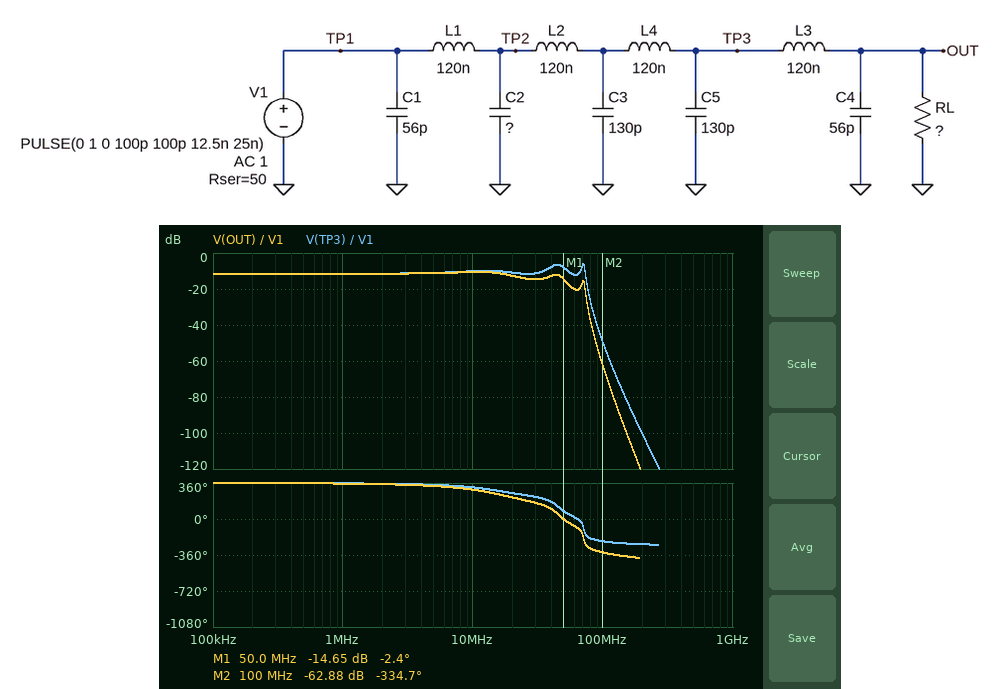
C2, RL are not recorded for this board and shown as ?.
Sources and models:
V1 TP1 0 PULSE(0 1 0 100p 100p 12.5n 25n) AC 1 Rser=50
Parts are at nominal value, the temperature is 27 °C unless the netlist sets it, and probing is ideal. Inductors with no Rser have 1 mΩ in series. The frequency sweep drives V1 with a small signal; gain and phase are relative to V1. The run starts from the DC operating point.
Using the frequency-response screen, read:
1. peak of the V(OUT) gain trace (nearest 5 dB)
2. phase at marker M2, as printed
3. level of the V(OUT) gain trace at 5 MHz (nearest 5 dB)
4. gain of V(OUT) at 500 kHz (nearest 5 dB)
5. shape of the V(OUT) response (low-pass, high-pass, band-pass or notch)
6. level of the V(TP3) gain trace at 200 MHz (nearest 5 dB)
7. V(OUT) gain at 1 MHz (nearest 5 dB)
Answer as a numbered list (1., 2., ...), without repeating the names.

1. -10 dB
2. -334.7 deg
3. -10 dB
4. -10 dB
5. low-pass
6. -100 dB
7. -10 dB
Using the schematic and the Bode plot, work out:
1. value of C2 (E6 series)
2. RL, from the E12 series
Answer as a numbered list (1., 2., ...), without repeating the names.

1. 330 pF
2. 18 Ω
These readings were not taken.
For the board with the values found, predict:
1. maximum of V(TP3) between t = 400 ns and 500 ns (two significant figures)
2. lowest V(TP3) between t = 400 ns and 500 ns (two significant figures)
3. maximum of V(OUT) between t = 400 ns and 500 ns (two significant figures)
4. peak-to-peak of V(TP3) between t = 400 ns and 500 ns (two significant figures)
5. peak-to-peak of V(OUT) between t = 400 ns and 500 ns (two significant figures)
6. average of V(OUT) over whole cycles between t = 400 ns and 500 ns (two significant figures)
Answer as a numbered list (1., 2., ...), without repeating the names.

1. 390 mV
2. -130 mV
3. 280 mV
4. 520 mV
5. 290 mV
6. 130 mV
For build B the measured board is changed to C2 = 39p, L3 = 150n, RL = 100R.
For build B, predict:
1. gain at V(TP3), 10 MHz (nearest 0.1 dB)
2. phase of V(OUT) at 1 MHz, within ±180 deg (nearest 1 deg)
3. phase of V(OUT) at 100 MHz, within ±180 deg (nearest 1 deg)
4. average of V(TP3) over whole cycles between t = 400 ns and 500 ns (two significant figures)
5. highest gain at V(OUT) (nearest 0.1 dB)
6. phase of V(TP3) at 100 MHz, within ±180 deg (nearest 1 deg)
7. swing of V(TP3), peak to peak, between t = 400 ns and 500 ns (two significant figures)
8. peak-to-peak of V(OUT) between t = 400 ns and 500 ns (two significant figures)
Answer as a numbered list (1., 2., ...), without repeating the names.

1. -4.7 dB
2. -6 deg
3. 134 deg
4. 340 mV
5. -3.1 dB
6. -68 deg
7. 460 mV
8. 780 mV
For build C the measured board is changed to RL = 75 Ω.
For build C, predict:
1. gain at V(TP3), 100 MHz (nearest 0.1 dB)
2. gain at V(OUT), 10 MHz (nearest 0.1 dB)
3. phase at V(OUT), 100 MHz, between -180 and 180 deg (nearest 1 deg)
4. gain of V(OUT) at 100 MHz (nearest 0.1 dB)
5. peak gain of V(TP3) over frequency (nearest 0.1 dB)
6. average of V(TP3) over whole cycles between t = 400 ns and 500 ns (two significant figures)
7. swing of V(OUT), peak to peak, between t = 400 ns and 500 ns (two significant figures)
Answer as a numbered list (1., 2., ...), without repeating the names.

1. -49.0 dB
2. -6.9 dB
3. -11 deg
4. -54.7 dB
5. -4.4 dB
6. 300 mV
7. 430 mV
